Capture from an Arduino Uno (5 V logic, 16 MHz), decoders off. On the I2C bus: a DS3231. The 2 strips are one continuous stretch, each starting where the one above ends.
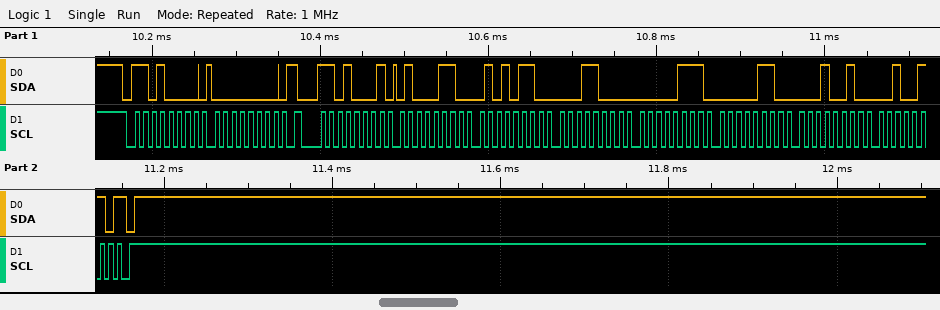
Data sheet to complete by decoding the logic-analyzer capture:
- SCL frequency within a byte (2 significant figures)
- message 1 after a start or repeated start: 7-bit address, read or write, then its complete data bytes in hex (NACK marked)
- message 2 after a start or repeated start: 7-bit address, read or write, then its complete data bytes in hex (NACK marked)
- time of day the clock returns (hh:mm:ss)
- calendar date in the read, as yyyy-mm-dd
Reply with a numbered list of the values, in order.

1. 100 kHz
2. 0x68 write: 00
3. 0x68 read: 46 56 18 07 06 12 26 NACK
4. 18:56:46
5. 2026-12-06
